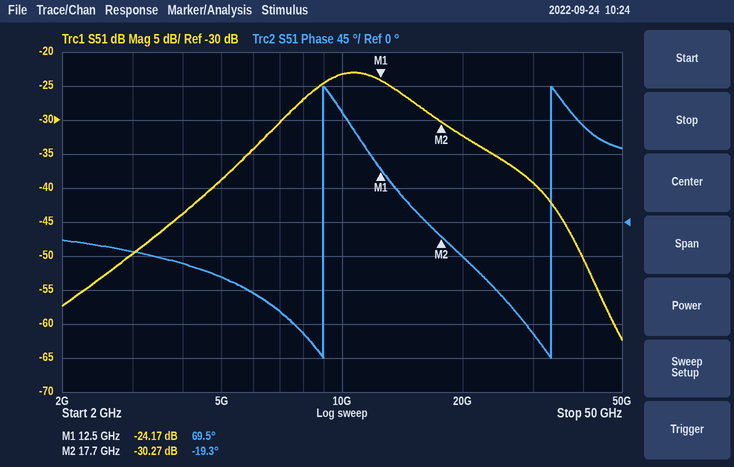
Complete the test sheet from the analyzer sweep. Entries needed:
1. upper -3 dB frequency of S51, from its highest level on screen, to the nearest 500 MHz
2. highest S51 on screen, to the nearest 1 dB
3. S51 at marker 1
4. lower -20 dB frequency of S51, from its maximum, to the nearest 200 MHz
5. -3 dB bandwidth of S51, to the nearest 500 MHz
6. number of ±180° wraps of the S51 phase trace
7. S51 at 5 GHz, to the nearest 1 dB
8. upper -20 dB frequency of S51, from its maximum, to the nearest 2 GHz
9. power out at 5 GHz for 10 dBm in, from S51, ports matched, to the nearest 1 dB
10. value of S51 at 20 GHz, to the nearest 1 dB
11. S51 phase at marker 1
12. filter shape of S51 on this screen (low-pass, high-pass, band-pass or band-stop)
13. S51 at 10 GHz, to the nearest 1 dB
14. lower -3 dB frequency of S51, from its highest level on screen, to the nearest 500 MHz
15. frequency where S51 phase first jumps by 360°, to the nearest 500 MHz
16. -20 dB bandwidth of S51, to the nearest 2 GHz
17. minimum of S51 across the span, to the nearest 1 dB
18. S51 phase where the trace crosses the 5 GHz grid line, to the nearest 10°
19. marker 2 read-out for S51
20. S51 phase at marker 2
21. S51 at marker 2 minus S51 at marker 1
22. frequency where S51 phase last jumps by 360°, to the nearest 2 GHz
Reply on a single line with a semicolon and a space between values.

14.0 GHz; -23 dB; -24.17 dB; 4.2 GHz; 5.5 GHz; 2; -39 dB; 34 GHz; -29 dBm; -32 dB; 69.5°; band-pass; -23 dB; 8.5 GHz; 9.0 GHz; 30 GHz; -62 dB; -70°; -30.27 dB; -19.3°; -6.10 dB; 34 GHz
